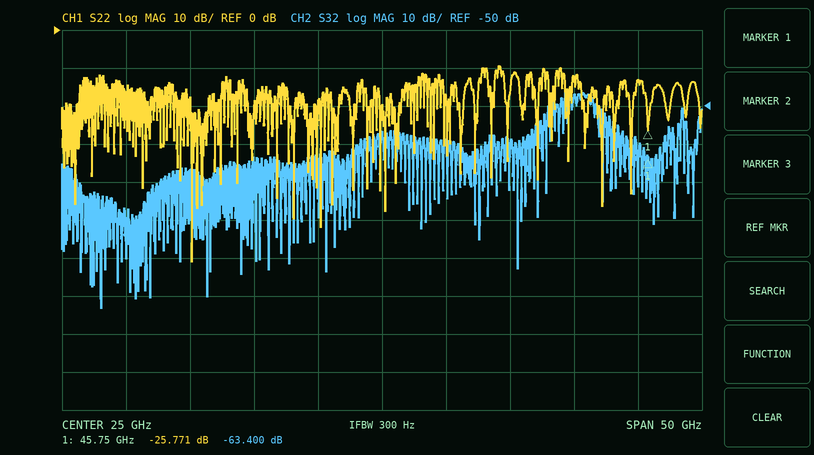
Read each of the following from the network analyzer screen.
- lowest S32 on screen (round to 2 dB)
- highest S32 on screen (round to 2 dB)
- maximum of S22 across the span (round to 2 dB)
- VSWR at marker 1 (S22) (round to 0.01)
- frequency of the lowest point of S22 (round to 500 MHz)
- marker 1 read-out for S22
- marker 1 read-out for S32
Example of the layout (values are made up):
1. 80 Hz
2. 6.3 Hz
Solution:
1. -104 dB
2. -46 dB
3. -10 dB
4. 1.11
5. 10.0 GHz
6. -25.771 dB
7. -63.400 dB
